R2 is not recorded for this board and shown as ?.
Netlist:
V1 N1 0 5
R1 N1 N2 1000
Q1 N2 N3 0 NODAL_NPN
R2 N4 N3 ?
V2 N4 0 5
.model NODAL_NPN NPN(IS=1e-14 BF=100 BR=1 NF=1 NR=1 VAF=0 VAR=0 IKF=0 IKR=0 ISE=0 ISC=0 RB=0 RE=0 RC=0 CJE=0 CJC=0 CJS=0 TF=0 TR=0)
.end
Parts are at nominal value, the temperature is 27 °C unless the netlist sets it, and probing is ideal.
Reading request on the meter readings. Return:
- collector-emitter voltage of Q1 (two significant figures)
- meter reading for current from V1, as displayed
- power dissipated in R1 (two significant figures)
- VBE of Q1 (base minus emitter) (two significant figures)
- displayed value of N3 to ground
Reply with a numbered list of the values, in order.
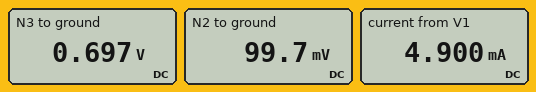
1. 100 mV
2. 4.900 mA
3. 24 mW
4. 700 mV
5. 0.697 V
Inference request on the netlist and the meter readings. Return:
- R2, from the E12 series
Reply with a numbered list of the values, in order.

1. 27 kΩ
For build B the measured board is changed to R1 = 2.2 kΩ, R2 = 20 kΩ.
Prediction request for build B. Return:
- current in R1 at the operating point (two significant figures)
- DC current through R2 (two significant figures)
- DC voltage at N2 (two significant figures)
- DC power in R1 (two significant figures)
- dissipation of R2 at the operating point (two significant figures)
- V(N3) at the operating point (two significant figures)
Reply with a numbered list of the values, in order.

1. 2.2 mA
2. 220 µA
3. 68 mV
4. 11 mW
5. 930 µW
6. 680 mV
